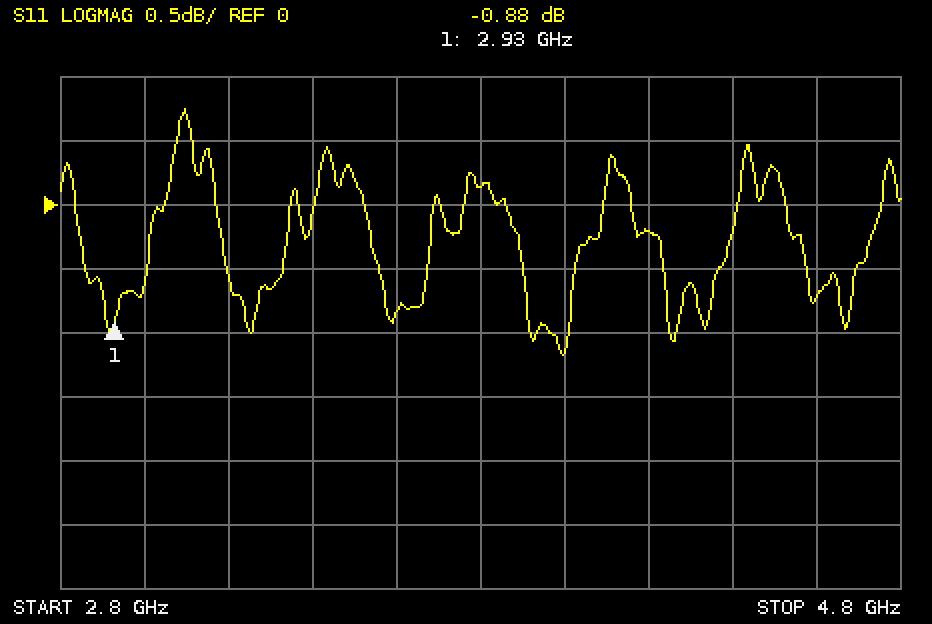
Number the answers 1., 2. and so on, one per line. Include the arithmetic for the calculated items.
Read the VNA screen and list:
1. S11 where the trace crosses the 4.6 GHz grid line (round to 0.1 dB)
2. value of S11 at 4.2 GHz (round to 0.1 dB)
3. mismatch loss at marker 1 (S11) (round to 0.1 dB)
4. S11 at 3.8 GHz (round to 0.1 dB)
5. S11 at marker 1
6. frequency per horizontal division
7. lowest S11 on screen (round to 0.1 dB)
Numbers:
1. -0.7 dB
2. -0.2 dB
3. −10 log10(1 − 10^(-0.88/10)) ≈ 7.4 dB
4. 0.1 dB
5. -0.88 dB
6. 200 MHz
7. -1.2 dB
